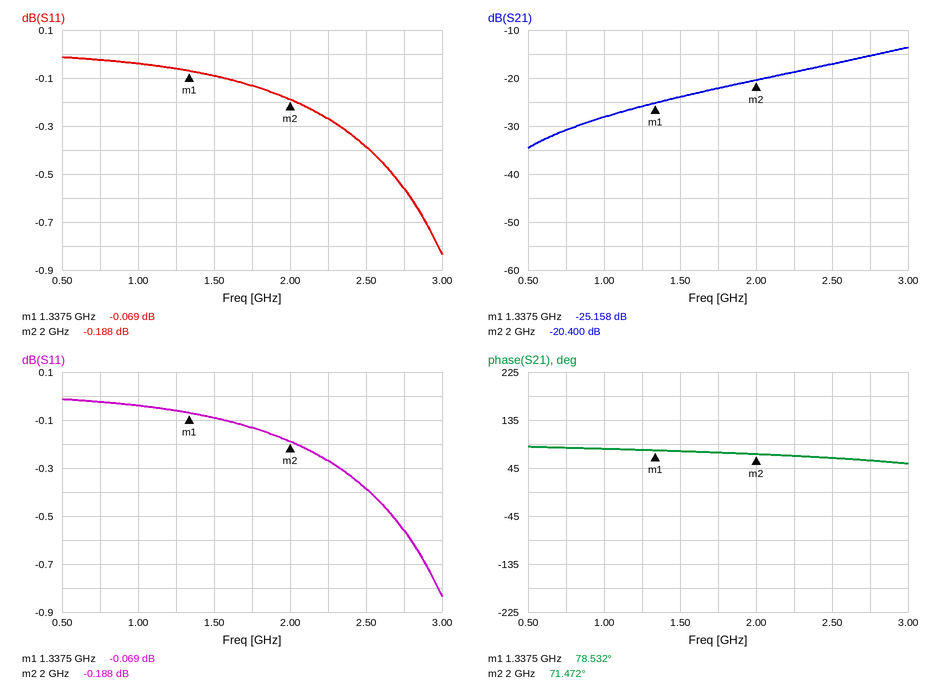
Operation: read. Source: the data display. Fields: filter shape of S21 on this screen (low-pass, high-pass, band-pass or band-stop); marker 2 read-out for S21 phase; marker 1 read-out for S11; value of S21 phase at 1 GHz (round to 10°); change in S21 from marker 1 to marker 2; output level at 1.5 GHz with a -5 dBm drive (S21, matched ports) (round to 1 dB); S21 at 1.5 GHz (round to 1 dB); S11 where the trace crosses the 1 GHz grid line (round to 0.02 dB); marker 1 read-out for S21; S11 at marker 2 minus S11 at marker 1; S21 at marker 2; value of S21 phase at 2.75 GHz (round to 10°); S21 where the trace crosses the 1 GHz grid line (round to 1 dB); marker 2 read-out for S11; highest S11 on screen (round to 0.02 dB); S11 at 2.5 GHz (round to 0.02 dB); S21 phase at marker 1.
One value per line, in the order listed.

high-pass
71.472°
-0.069 dB
80°
4.758 dB
-29 dBm
-24 dB
-0.04 dB
-25.158 dB
-0.119 dB
-20.400 dB
60°
-28 dB
-0.188 dB
-0.02 dB
-0.38 dB
78.532°
